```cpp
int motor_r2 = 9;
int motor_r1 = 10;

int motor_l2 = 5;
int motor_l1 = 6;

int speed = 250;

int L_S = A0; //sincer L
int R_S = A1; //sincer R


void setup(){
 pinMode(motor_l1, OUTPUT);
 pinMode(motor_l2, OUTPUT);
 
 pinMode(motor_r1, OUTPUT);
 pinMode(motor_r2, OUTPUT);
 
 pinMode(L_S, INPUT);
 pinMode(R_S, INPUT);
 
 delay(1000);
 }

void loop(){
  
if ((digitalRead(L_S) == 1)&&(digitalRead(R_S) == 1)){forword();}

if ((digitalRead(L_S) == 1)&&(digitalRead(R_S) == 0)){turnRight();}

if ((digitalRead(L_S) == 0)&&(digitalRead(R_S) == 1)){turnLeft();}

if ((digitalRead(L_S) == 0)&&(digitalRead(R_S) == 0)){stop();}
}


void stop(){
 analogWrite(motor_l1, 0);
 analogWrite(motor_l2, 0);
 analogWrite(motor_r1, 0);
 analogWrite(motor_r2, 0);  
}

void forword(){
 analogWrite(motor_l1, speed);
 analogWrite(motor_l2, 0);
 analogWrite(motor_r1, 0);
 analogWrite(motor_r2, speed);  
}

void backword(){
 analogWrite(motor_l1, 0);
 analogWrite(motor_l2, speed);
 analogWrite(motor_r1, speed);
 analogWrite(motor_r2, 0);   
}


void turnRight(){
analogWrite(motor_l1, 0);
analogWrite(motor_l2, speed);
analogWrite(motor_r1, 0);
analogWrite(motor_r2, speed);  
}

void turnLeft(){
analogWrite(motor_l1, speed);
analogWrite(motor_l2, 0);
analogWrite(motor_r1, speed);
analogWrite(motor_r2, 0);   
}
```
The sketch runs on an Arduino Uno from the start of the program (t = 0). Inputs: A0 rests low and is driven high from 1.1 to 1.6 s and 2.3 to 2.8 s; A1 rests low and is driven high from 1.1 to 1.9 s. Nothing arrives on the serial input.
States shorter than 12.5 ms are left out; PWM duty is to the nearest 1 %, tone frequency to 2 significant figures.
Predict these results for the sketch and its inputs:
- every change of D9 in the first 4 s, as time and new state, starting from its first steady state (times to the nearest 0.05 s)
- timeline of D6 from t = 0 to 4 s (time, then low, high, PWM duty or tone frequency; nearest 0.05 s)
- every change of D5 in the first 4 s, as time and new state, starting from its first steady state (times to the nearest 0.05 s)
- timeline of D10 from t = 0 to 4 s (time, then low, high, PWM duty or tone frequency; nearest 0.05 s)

0 s low; 1.1 s PWM 98 %; 1.6 s low; 2.3 s PWM 98 %; 2.8 s low
0 s low; 1.1 s PWM 98 %; 1.9 s low
0 s low; 2.3 s PWM 98 %; 2.8 s low
0 s low; 1.6 s PWM 98 %; 1.9 s low
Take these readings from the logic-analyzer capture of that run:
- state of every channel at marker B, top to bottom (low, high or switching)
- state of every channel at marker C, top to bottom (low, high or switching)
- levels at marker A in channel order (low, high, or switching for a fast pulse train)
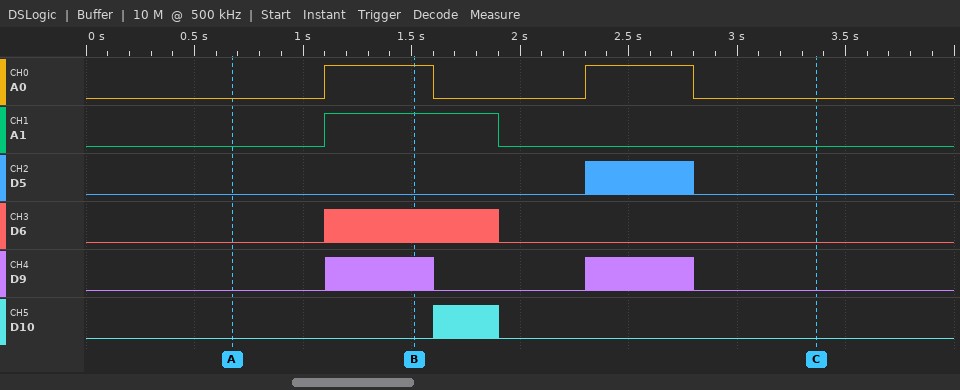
A0 high, A1 high, D5 low, D6 switching, D9 switching, D10 low
A0 low, A1 low, D5 low, D6 low, D9 low, D10 low
A0 low, A1 low, D5 low, D6 low, D9 low, D10 low
